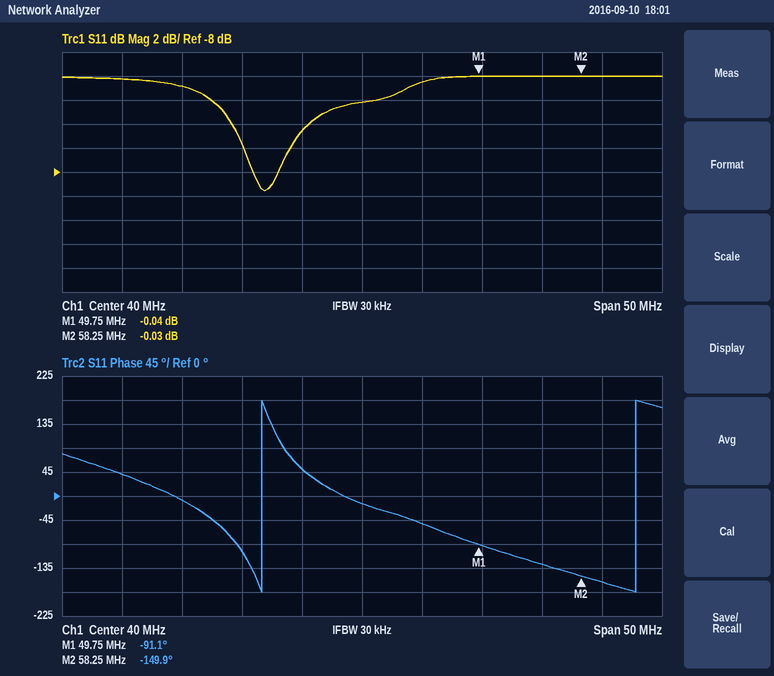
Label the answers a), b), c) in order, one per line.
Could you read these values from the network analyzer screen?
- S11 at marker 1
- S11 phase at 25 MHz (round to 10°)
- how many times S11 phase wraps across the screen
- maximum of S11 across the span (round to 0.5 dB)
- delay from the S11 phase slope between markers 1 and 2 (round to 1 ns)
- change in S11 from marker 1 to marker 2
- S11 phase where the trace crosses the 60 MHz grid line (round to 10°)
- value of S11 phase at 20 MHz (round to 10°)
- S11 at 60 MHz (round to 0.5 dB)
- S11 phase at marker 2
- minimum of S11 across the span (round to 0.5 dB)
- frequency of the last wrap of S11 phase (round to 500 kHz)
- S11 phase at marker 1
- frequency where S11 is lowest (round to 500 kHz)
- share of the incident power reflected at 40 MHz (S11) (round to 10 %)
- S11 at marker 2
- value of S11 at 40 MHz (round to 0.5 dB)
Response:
a) -0.04 dB
b) -10°
c) 2
d) 0.0 dB
e) 19 ns
f) 0.01 dB
g) -160°
h) 40°
i) 0.0 dB
j) -149.9°
k) -9.5 dB
l) 63.0 MHz
m) -91.1°
n) 32.0 MHz
o) 60 %
p) -0.03 dB
q) -2.0 dB
